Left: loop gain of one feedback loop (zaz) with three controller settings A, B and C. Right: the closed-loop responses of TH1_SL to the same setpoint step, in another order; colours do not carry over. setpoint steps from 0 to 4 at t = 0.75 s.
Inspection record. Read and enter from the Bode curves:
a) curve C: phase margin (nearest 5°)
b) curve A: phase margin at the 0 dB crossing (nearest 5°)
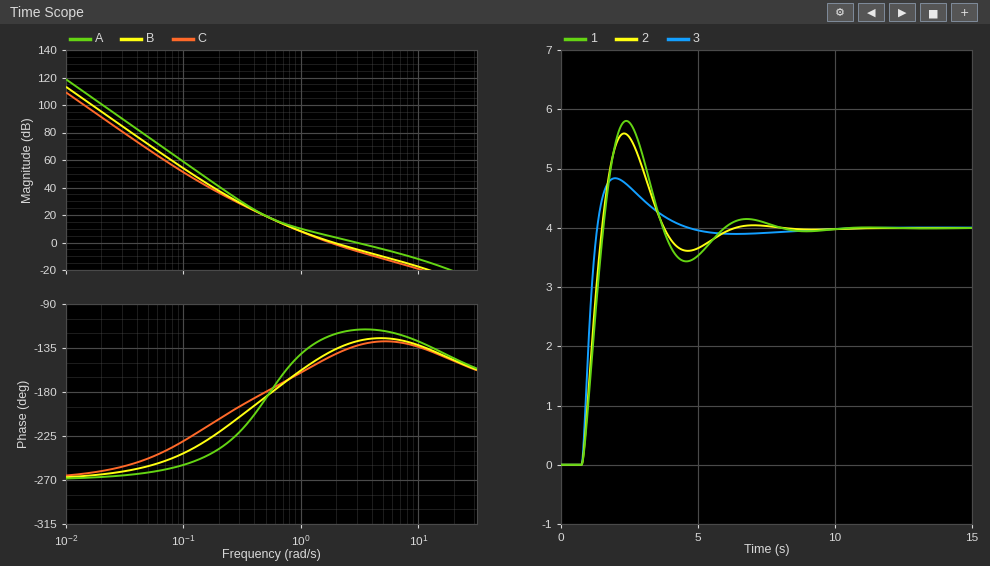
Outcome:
35°
65°
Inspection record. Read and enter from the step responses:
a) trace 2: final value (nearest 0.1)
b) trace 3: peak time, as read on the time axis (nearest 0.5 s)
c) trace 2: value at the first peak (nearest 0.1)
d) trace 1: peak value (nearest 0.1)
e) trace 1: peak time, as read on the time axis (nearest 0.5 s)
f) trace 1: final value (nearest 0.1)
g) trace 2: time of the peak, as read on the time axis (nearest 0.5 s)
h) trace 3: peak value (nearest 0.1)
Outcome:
4.0
2.0 s
5.6
5.8
2.5 s
4.0
2.5 s
4.8
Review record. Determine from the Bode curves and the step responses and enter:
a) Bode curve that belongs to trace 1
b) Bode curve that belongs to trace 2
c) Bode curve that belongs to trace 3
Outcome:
C
B
A
